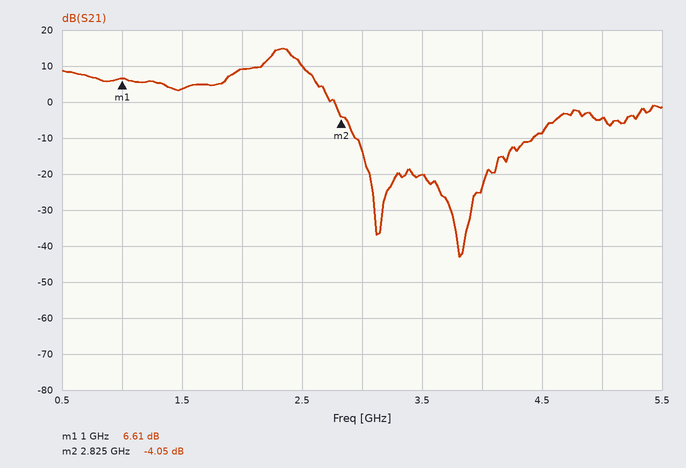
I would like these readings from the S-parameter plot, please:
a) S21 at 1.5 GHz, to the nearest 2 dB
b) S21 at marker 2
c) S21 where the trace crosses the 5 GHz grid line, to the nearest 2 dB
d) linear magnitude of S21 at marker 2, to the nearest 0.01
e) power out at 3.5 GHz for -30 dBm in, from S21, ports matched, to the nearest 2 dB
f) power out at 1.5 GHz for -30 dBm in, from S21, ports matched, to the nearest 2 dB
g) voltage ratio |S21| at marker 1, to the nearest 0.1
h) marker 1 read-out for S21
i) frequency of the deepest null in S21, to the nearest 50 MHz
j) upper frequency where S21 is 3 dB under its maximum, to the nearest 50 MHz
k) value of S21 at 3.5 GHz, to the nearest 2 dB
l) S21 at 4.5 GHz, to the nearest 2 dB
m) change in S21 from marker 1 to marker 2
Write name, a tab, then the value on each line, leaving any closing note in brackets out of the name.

S21 at 1.5 GHz, to the nearest 2 dB	4 dB
S21 at marker 2	-4.05 dB
S21 where the trace crosses the 5 GHz grid line, to the nearest 2 dB	-4 dB
linear magnitude of S21 at marker 2, to the nearest 0.01	0.63
power out at 3.5 GHz for -30 dBm in, from S21, ports matched, to the nearest 2 dB	-50 dBm
power out at 1.5 GHz for -30 dBm in, from S21, ports matched, to the nearest 2 dB	-26 dBm
voltage ratio |S21| at marker 1, to the nearest 0.1	2.1
marker 1 read-out for S21	6.61 dB
frequency of the deepest null in S21, to the nearest 50 MHz	3.80 GHz
upper frequency where S21 is 3 dB under its maximum, to the nearest 50 MHz	2.45 GHz
value of S21 at 3.5 GHz, to the nearest 2 dB	-20 dB
S21 at 4.5 GHz, to the nearest 2 dB	-8 dB
change in S21 from marker 1 to marker 2	-10.66 dB
